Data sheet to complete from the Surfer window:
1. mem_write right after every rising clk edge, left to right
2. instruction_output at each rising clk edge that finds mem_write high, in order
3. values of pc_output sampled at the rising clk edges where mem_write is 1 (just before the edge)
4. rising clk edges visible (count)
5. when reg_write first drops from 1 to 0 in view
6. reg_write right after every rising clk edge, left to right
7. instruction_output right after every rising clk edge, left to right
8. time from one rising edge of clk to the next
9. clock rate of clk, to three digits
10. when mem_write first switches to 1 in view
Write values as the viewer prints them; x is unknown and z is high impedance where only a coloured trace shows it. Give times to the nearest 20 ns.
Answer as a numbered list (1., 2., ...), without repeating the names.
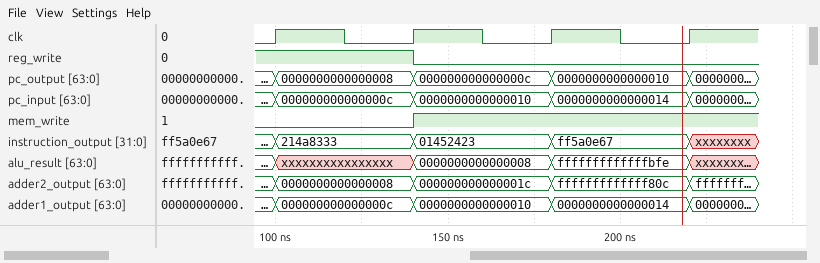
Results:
1. 0 1 1 1
2. 01452423, ff5a0e67
3. 000000000000000c, 0000000000000010
4. 4
5. 140 ns
6. 1 0 0 0
7. 214a8333, 01452423, ff5a0e67, xxxxxxxx
8. 40 ns
9. 25.0 MHz
10. 140 ns
